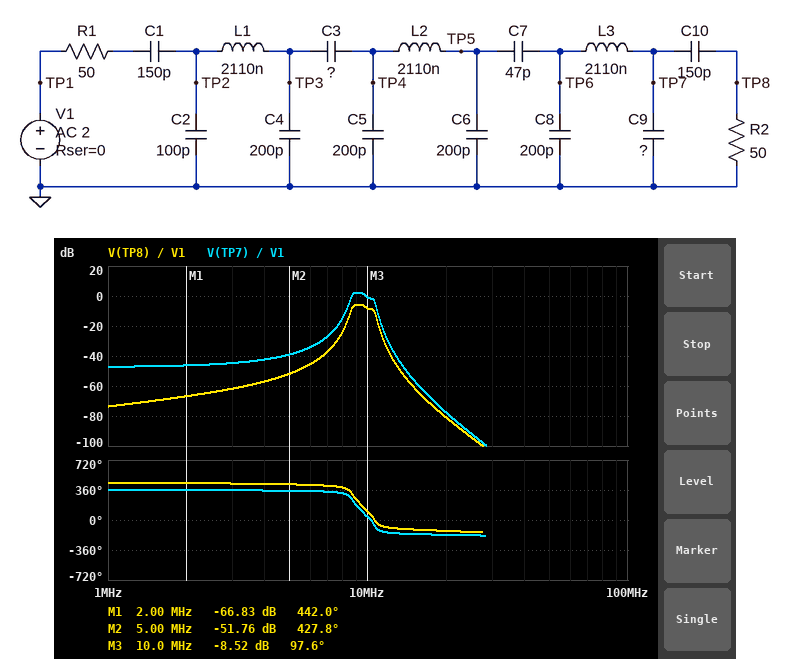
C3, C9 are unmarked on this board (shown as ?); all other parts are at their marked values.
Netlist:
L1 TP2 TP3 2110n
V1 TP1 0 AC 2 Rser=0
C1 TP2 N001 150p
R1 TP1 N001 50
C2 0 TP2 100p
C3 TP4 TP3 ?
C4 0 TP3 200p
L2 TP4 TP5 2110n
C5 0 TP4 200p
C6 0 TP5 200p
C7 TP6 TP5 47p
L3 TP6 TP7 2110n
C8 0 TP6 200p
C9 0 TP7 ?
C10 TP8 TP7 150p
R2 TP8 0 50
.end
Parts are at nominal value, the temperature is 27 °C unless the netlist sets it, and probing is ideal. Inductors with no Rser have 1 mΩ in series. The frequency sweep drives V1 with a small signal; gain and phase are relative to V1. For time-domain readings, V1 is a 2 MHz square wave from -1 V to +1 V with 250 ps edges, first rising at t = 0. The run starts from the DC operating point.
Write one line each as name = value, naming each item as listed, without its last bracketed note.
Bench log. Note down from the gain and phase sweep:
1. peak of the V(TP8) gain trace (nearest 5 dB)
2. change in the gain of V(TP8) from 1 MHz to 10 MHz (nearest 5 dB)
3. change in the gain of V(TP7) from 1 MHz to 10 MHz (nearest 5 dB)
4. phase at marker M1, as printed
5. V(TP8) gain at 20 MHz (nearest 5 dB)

peak of the V(TP8) gain trace = -5 dB
change in the gain of V(TP8) from 1 MHz to 10 MHz = 65 dB
change in the gain of V(TP7) from 1 MHz to 10 MHz = 45 dB
phase at marker M1, as printed = 442.0 deg
V(TP8) gain at 20 MHz = -80 dB
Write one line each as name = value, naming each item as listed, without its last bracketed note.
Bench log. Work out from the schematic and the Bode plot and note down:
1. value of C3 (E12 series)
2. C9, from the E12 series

value of C3 = 100 pF
C9, from the E12 series = 180 pF
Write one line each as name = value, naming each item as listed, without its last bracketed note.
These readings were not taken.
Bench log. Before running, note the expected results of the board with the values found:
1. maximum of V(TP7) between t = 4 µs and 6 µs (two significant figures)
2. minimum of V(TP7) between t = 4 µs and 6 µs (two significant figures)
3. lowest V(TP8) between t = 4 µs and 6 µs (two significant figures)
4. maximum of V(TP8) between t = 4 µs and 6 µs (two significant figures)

maximum of V(TP7) between t = 4 µs and 6 µs = 240 mV
minimum of V(TP7) between t = 4 µs and 6 µs = -230 mV
lowest V(TP8) between t = 4 µs and 6 µs = -97 mV
maximum of V(TP8) between t = 4 µs and 6 µs = 97 mV
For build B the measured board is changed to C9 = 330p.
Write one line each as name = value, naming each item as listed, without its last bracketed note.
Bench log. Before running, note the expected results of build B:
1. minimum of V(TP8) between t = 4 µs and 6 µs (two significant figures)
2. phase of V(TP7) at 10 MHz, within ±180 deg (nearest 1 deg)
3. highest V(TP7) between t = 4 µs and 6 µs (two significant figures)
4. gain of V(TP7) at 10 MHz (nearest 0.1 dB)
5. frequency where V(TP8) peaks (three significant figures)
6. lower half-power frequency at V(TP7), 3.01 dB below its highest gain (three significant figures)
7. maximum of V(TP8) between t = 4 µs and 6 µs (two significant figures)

minimum of V(TP8) between t = 4 µs and 6 µs = -47 mV
phase of V(TP7) at 10 MHz, within ±180 deg = 2 deg
highest V(TP7) between t = 4 µs and 6 µs = 120 mV
gain of V(TP7) at 10 MHz = -7.7 dB
frequency where V(TP8) peaks = 8.45 MHz
lower half-power frequency at V(TP7), 3.01 dB below its highest gain = 8.29 MHz
maximum of V(TP8) between t = 4 µs and 6 µs = 47 mV
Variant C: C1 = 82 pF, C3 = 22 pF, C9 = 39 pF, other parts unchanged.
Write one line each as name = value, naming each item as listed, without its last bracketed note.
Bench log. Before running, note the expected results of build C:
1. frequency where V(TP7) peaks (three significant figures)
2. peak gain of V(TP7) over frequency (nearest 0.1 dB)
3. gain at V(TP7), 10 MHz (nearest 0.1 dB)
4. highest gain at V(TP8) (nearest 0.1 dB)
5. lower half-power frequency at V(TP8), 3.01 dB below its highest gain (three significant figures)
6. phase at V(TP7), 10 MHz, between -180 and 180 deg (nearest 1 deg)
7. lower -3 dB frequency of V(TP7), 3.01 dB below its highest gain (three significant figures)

frequency where V(TP7) peaks = 10.1 MHz
peak gain of V(TP7) over frequency = -1.6 dB
gain at V(TP7), 10 MHz = -3.4 dB
highest gain at V(TP8) = -8.9 dB
lower half-power frequency at V(TP8), 3.01 dB below its highest gain = 9.97 MHz
phase at V(TP7), 10 MHz, between -180 and 180 deg = -120 deg
lower -3 dB frequency of V(TP7), 3.01 dB below its highest gain = 9.96 MHz
